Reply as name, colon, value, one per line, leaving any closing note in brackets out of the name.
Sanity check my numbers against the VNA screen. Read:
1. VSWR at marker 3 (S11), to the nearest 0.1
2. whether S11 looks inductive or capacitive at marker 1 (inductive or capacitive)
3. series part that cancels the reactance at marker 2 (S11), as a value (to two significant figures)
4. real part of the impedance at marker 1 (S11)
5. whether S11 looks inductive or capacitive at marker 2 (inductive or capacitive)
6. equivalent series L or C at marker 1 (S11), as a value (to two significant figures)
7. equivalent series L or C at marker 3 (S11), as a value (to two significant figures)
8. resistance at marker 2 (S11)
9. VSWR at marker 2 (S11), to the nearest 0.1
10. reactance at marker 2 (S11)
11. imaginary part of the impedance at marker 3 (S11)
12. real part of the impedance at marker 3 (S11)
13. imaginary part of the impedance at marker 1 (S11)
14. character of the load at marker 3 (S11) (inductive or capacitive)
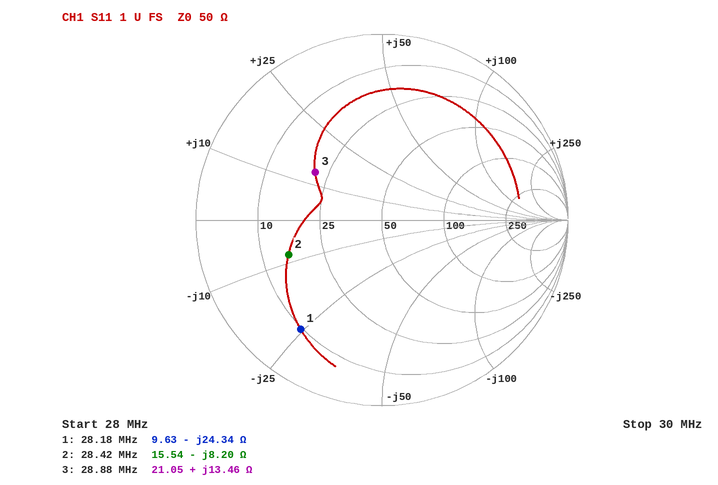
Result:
VSWR at marker 3 (S11), to the nearest 0.1: 2.6
whether S11 looks inductive or capacitive at marker 1: capacitive
series part that cancels the reactance at marker 2 (S11), as a value: 46 nH
real part of the impedance at marker 1: 9.63 Ω
whether S11 looks inductive or capacitive at marker 2: capacitive
equivalent series L or C at marker 1 (S11), as a value: 230 pF
equivalent series L or C at marker 3 (S11), as a value: 74 nH
resistance at marker 2: 15.54 Ω
VSWR at marker 2 (S11), to the nearest 0.1: 3.3
reactance at marker 2: -8.20 Ω
imaginary part of the impedance at marker 3: +13.46 Ω
real part of the impedance at marker 3: 21.05 Ω
imaginary part of the impedance at marker 1: -24.34 Ω
character of the load at marker 3 (S11): inductive
